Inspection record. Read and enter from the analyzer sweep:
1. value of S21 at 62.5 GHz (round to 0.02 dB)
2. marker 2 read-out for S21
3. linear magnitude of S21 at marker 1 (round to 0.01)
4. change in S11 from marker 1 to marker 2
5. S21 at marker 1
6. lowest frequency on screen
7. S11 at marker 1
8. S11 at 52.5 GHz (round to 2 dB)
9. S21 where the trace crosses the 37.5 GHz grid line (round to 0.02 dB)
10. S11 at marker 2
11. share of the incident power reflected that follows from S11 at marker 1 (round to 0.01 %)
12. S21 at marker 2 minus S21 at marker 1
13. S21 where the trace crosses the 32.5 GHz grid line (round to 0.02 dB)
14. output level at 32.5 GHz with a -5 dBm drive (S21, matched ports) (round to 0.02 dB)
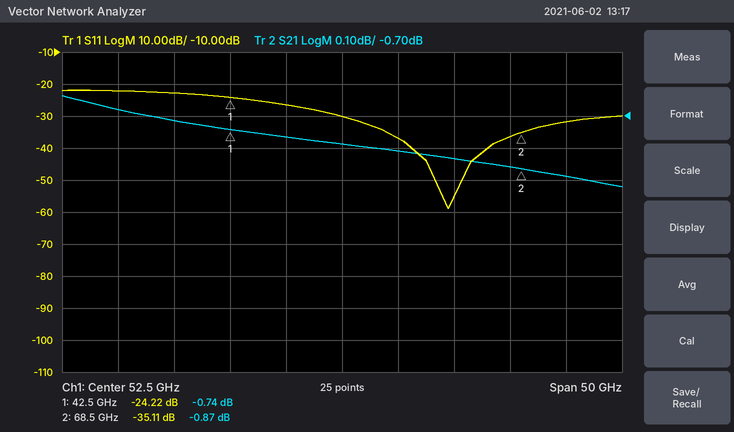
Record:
-0.84 dB
-0.87 dB
0.92
-10.89 dB
-0.74 dB
27.5 GHz
-24.22 dB
-30 dB
-0.72 dB
-35.11 dB
0.38 %
-0.13 dB
-0.68 dB
-5.68 dBm
